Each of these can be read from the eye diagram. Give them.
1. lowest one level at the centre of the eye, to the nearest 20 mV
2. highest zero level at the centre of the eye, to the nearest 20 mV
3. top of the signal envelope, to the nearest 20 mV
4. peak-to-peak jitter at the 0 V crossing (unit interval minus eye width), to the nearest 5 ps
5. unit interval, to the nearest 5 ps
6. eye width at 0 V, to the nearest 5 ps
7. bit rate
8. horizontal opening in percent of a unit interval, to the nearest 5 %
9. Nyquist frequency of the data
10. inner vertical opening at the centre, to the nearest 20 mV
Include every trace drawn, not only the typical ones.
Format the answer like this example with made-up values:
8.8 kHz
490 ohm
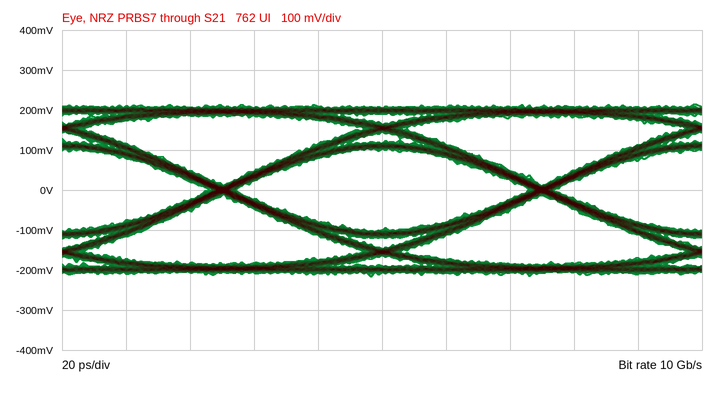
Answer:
100 mV
-100 mV
220 mV
10 ps
100 ps
90 ps
10 Gb/s
90 %
5 GHz
200 mV
